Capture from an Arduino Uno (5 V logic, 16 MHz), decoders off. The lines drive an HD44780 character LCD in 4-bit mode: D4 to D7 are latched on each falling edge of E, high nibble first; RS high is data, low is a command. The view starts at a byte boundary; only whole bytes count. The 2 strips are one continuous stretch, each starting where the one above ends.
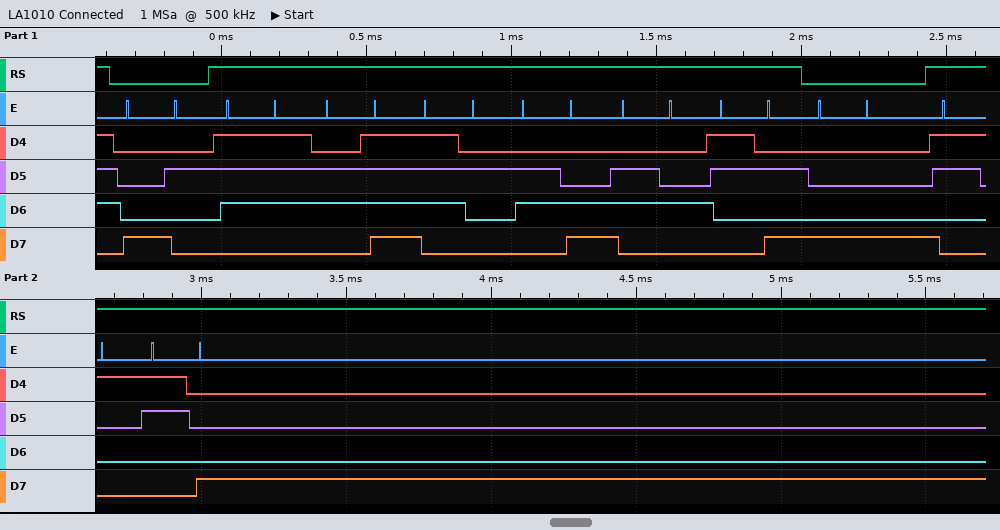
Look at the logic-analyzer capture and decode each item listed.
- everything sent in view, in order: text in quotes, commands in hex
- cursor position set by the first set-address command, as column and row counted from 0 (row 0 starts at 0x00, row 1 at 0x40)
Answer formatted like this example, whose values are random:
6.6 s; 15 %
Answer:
0x82 "world:" 0x88 "18"; column 2, row 0
